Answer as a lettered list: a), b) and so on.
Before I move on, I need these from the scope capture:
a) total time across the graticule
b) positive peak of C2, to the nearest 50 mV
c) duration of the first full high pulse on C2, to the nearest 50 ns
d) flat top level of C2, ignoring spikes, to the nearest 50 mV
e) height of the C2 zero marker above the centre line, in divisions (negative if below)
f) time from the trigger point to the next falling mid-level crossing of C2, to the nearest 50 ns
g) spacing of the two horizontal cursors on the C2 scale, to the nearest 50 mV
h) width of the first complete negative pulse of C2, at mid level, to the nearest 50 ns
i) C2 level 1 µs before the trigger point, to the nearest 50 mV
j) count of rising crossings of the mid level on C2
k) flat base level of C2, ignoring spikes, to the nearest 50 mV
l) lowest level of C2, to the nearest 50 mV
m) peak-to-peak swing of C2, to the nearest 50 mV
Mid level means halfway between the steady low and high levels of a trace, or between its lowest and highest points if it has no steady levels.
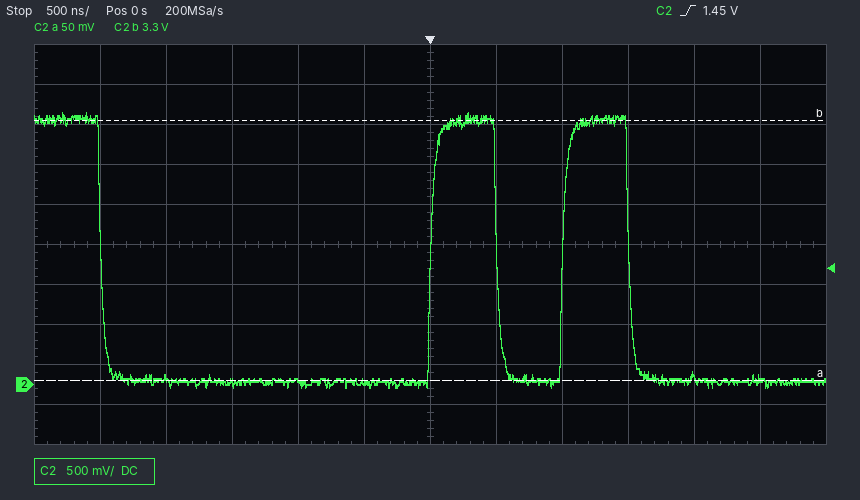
a) 6 µs
b) 3.40 V
c) 500 ns
d) 3.30 V
e) -3.5 div
f) 500 ns
g) 3.25 V
h) 2.50 µs
i) 50 mV
j) 2
k) 50 mV
l) -50 mV
m) 3.45 V
